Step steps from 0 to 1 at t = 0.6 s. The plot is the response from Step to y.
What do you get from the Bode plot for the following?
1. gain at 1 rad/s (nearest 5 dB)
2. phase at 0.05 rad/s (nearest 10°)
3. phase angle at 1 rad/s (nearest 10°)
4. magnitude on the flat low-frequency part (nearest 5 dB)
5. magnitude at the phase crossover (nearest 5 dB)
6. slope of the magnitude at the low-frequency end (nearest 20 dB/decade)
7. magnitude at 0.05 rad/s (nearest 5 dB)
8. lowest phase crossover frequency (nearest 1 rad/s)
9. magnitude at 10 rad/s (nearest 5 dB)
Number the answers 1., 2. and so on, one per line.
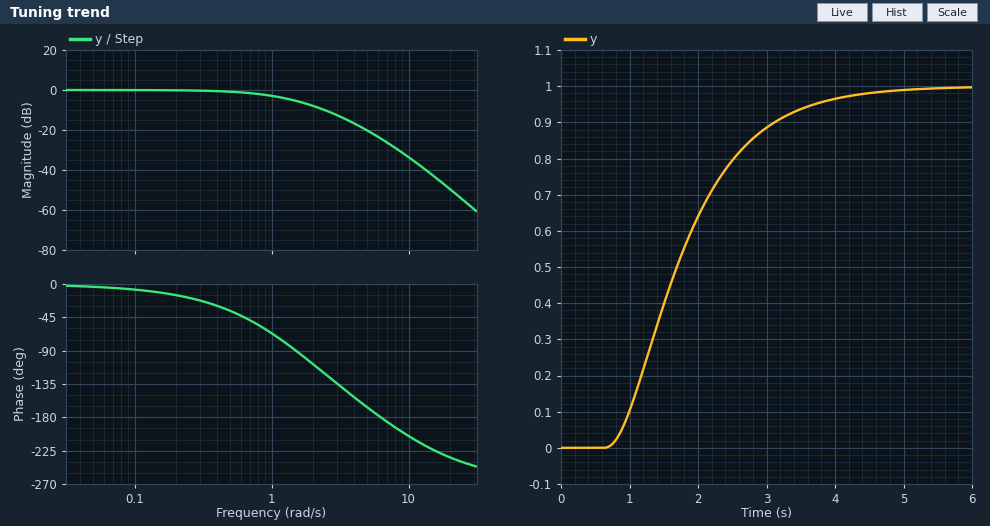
1. -5 dB
2. 0°
3. -70°
4. 0 dB
5. -25 dB
6. 0 dB/decade
7. 0 dB
8. 6 rad/s
9. -35 dB
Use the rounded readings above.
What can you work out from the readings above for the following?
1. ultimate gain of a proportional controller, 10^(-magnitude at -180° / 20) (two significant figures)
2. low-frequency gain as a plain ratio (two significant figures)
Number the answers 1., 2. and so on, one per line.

1. 18
2. 1.0
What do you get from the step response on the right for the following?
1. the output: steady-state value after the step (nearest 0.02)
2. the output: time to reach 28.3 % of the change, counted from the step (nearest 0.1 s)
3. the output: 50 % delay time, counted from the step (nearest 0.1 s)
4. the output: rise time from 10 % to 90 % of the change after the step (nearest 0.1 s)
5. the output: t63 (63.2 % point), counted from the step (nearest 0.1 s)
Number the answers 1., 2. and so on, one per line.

1. 1.00
2. 0.7 s
3. 1.1 s
4. 2.1 s
5. 1.4 s
